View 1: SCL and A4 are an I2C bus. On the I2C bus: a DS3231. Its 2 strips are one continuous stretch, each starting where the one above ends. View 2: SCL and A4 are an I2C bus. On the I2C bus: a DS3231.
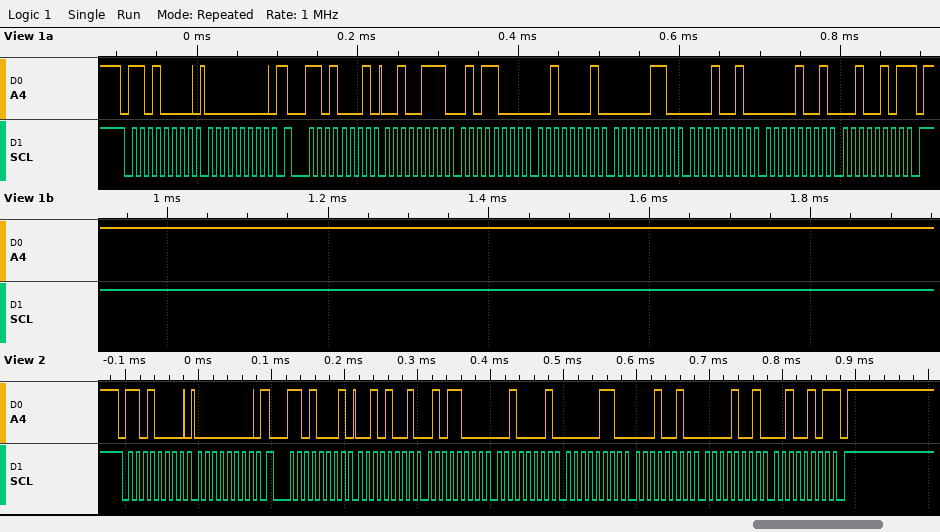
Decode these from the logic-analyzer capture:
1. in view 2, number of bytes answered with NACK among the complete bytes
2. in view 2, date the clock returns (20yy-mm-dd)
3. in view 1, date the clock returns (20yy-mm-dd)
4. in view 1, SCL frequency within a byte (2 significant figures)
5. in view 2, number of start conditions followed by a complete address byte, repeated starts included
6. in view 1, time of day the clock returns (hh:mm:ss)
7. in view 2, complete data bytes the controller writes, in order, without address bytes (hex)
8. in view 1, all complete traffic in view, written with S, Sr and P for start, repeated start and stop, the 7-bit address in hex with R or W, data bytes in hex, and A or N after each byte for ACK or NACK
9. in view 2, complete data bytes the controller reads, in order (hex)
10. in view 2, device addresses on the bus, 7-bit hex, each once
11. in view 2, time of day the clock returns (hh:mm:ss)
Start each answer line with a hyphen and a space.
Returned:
- 1
- 2025-09-12
- 2025-09-12
- 100 kHz
- 2
- 21:58:27
- 00
- S 68W A 00 A Sr 68R A 27 A 58 A 21 A 06 A 12 A 09 A 25 N P
- 29 58 21 06 12 09 25
- 0x68
- 21:58:29
